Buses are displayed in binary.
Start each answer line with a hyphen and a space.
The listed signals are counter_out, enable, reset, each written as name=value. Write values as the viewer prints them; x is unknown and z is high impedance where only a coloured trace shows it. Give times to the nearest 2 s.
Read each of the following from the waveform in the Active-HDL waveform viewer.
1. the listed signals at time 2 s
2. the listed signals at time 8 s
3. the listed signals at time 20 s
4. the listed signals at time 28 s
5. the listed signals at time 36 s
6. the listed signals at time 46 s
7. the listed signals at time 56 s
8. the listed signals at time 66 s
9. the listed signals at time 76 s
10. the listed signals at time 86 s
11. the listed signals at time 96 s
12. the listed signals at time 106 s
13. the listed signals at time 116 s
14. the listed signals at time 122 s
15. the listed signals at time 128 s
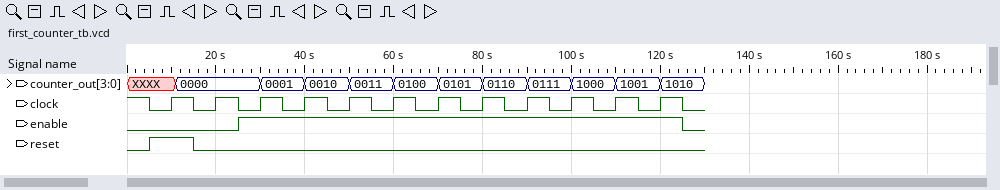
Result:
- counter_out=XXXX, enable=0, reset=0
- counter_out=XXXX, enable=0, reset=1
- counter_out=0000, enable=0, reset=0
- counter_out=0000, enable=1, reset=0
- counter_out=0001, enable=1, reset=0
- counter_out=0010, enable=1, reset=0
- counter_out=0011, enable=1, reset=0
- counter_out=0100, enable=1, reset=0
- counter_out=0101, enable=1, reset=0
- counter_out=0110, enable=1, reset=0
- counter_out=0111, enable=1, reset=0
- counter_out=1000, enable=1, reset=0
- counter_out=1001, enable=1, reset=0
- counter_out=1010, enable=1, reset=0
- counter_out=1010, enable=0, reset=0
